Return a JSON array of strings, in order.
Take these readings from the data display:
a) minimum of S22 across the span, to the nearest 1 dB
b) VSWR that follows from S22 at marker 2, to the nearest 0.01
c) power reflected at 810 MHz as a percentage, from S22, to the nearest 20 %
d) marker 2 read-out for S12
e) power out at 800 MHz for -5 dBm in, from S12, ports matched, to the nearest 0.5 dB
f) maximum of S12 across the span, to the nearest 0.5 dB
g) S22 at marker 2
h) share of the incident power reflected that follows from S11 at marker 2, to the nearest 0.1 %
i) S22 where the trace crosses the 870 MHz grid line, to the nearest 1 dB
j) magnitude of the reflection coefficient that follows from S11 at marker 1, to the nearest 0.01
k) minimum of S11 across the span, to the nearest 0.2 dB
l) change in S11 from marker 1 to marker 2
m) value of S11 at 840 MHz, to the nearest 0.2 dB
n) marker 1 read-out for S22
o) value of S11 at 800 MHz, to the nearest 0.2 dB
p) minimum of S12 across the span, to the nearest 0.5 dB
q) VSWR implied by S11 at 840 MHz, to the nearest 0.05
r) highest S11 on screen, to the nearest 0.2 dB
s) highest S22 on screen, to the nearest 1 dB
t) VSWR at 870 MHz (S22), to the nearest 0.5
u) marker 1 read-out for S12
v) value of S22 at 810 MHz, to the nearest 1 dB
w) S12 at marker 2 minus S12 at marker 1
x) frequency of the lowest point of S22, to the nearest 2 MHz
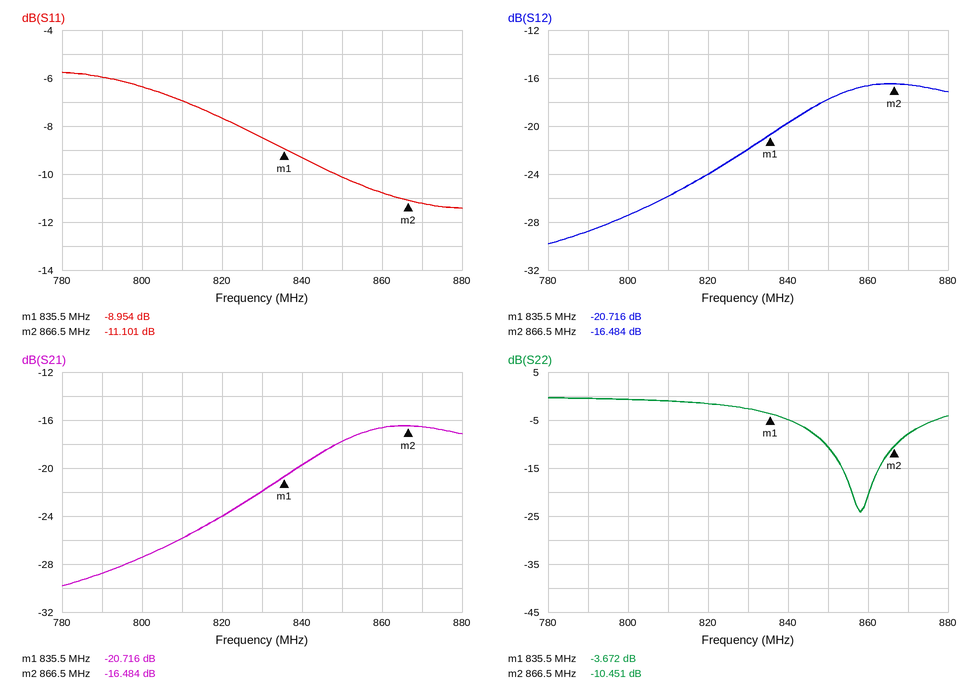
["-24 dB", "1.86", "80 %", "-16.484 dB", "-32.5 dBm", "-16.5 dB", "-10.451 dB", "7.8 %", "-8 dB", "0.36", "-11.4 dB", "-2.147 dB", "-9.4 dB", "-3.672 dB", "-6.4 dB", "-30.0 dB", "2.05", "-5.8 dB", "0 dB", "2.5", "-20.716 dB", "-1 dB", "4.232 dB", "858 MHz"]
